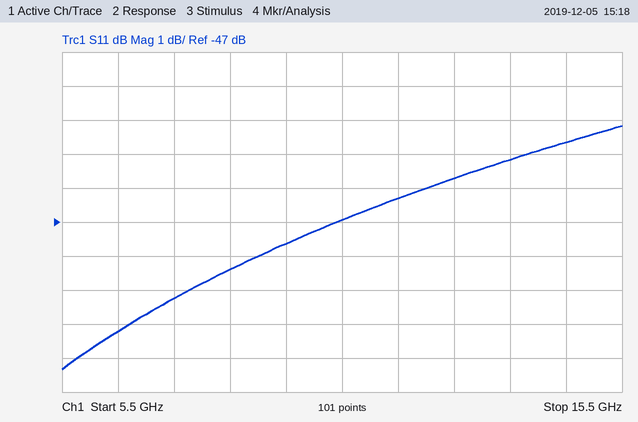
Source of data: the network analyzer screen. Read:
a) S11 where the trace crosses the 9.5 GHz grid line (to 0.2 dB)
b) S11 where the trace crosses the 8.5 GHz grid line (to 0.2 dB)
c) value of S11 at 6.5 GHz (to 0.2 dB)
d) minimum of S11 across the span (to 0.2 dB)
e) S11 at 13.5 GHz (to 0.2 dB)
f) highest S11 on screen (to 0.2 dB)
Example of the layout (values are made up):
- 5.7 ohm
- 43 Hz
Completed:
- -47.6 dB
- -48.4 dB
- -50.2 dB
- -51.4 dB
- -45.2 dB
- -44.2 dB
